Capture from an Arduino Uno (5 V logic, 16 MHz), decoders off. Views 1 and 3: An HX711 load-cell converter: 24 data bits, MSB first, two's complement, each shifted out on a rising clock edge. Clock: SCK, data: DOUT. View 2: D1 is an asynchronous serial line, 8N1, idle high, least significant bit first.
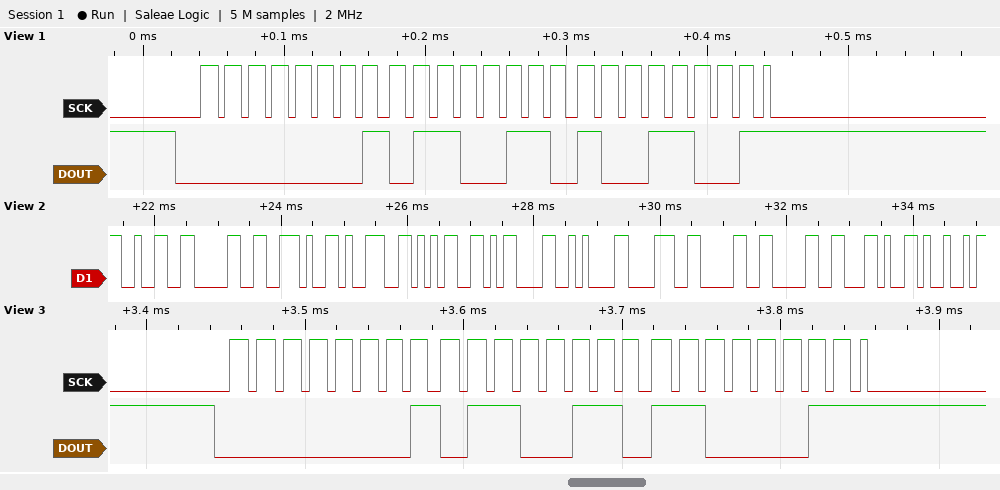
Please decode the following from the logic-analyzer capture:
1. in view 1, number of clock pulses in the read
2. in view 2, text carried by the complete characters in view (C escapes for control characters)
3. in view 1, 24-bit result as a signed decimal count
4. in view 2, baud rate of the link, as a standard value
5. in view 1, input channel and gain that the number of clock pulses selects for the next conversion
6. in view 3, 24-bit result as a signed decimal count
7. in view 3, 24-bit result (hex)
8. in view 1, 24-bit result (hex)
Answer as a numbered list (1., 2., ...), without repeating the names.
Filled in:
1. 25
2. "20.95\r\n800,I"
3. 91801
4. 9600 baud
5. channel A, gain 128
6. 91843
7. 0x0166C3
8. 0x016699
